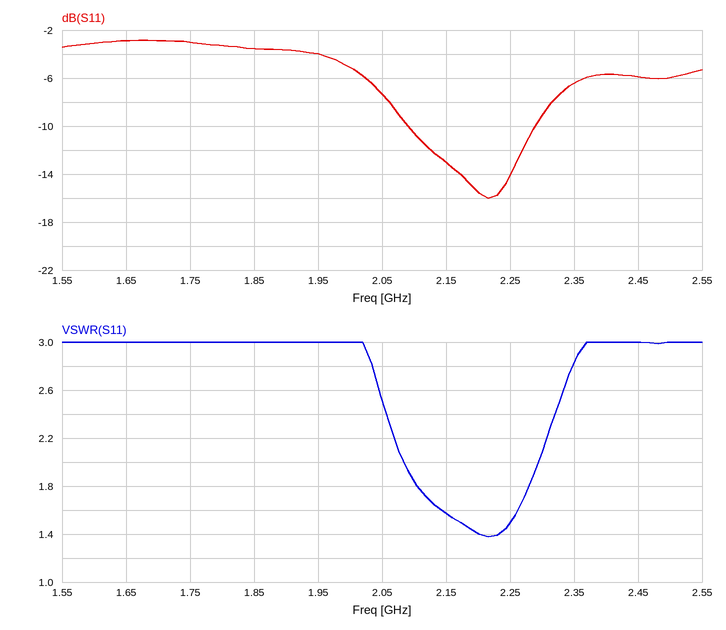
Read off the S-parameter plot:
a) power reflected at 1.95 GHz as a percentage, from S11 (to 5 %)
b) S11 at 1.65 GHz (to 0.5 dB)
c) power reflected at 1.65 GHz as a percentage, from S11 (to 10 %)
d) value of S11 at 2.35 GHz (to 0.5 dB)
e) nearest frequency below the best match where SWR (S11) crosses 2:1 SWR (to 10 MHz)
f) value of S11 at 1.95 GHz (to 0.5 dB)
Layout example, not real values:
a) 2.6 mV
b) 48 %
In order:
a) 40 %
b) -3.0 dB
c) 50 %
d) -6.5 dB
e) 2.08 GHz
f) -4.0 dB
